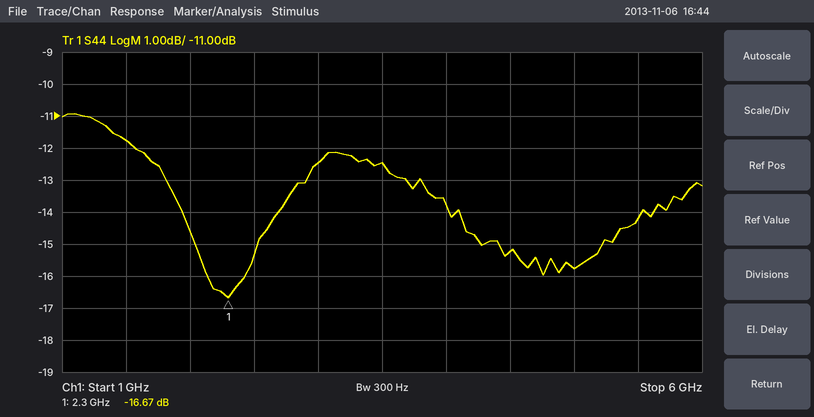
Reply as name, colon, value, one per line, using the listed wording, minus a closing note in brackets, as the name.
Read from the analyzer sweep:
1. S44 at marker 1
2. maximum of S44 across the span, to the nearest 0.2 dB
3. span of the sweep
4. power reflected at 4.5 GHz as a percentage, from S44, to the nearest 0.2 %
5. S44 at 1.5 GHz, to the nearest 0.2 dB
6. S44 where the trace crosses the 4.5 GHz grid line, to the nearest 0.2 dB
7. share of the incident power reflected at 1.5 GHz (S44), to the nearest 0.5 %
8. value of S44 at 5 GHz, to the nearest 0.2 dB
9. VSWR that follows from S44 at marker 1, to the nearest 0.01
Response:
S44 at marker 1: -16.67 dB
maximum of S44 across the span, to the nearest 0.2 dB: -11.0 dB
span of the sweep: 5 GHz
power reflected at 4.5 GHz as a percentage, from S44, to the nearest 0.2 %: 3.0 %
S44 at 1.5 GHz, to the nearest 0.2 dB: -11.8 dB
S44 where the trace crosses the 4.5 GHz grid line, to the nearest 0.2 dB: -15.2 dB
share of the incident power reflected at 1.5 GHz (S44), to the nearest 0.5 %: 6.5 %
value of S44 at 5 GHz, to the nearest 0.2 dB: -15.8 dB
VSWR that follows from S44 at marker 1, to the nearest 0.01: 1.34
